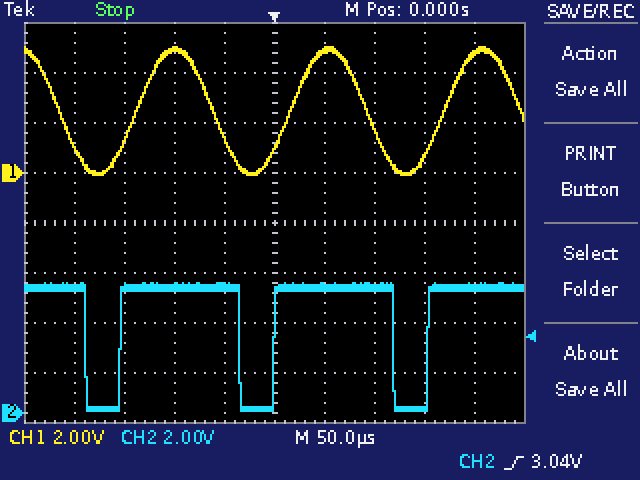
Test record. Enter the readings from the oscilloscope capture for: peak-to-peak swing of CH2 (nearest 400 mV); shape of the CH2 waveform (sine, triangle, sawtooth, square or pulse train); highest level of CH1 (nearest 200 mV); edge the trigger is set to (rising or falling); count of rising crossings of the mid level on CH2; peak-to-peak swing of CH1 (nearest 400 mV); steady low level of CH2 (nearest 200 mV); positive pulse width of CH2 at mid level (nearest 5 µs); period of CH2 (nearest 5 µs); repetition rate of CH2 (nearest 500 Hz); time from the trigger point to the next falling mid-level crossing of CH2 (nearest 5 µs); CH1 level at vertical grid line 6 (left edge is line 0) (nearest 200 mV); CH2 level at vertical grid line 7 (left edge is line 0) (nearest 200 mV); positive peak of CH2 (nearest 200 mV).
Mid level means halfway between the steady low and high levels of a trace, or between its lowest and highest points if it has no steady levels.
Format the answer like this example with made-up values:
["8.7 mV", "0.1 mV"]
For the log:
["5.2 V", "pulse train", "5.0 V", "rising", "3", "5.2 V", "200 mV", "120 µs", "155 µs", "6.5 kHz", "120 µs", "4.8 V", "5.0 V", "5.2 V"]
